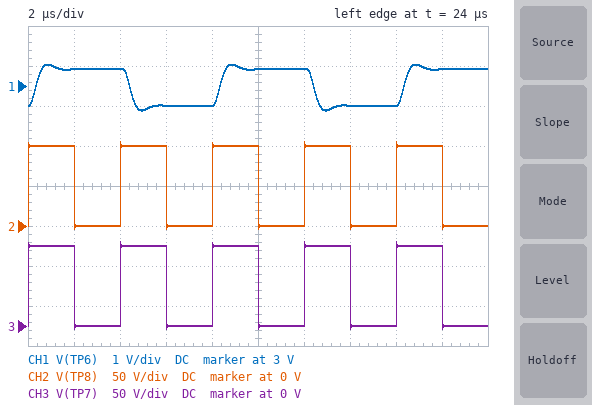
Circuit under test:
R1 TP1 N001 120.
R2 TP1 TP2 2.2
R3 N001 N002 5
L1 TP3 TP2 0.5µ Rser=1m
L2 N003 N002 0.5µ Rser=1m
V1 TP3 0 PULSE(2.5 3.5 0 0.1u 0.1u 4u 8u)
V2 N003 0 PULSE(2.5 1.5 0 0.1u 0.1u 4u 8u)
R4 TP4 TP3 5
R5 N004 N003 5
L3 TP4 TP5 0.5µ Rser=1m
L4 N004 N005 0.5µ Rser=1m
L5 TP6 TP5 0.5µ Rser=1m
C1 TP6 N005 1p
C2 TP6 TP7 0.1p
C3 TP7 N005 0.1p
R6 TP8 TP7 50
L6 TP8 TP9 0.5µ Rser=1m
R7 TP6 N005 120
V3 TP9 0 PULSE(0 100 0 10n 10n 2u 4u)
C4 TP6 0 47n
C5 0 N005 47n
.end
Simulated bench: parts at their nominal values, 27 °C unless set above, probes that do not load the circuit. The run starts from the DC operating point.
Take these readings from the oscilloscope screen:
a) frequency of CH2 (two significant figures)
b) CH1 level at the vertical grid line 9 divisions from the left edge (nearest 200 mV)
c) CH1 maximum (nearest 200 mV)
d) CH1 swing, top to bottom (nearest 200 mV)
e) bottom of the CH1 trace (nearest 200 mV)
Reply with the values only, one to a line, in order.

250 kHz
3.4 V
3.6 V
1.2 V
2.4 V
